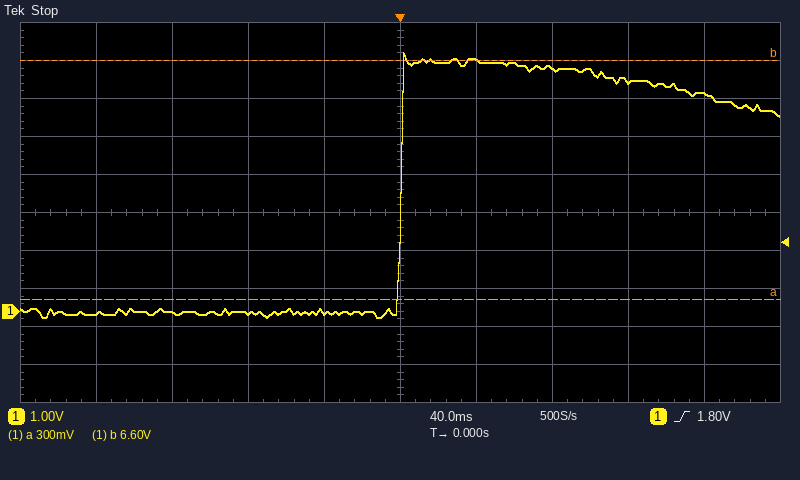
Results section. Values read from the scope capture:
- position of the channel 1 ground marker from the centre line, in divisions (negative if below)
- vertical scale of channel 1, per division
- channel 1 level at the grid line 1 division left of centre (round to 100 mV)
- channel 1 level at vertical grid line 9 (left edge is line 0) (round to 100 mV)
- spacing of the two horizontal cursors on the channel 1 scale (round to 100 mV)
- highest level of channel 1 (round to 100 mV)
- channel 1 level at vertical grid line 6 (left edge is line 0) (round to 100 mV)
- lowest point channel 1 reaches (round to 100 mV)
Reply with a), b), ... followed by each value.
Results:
a) -2.6 div
b) 1 V
c) 0.0 V
d) 5.7 V
e) 6.3 V
f) 6.8 V
g) 6.6 V
h) -200 mV
